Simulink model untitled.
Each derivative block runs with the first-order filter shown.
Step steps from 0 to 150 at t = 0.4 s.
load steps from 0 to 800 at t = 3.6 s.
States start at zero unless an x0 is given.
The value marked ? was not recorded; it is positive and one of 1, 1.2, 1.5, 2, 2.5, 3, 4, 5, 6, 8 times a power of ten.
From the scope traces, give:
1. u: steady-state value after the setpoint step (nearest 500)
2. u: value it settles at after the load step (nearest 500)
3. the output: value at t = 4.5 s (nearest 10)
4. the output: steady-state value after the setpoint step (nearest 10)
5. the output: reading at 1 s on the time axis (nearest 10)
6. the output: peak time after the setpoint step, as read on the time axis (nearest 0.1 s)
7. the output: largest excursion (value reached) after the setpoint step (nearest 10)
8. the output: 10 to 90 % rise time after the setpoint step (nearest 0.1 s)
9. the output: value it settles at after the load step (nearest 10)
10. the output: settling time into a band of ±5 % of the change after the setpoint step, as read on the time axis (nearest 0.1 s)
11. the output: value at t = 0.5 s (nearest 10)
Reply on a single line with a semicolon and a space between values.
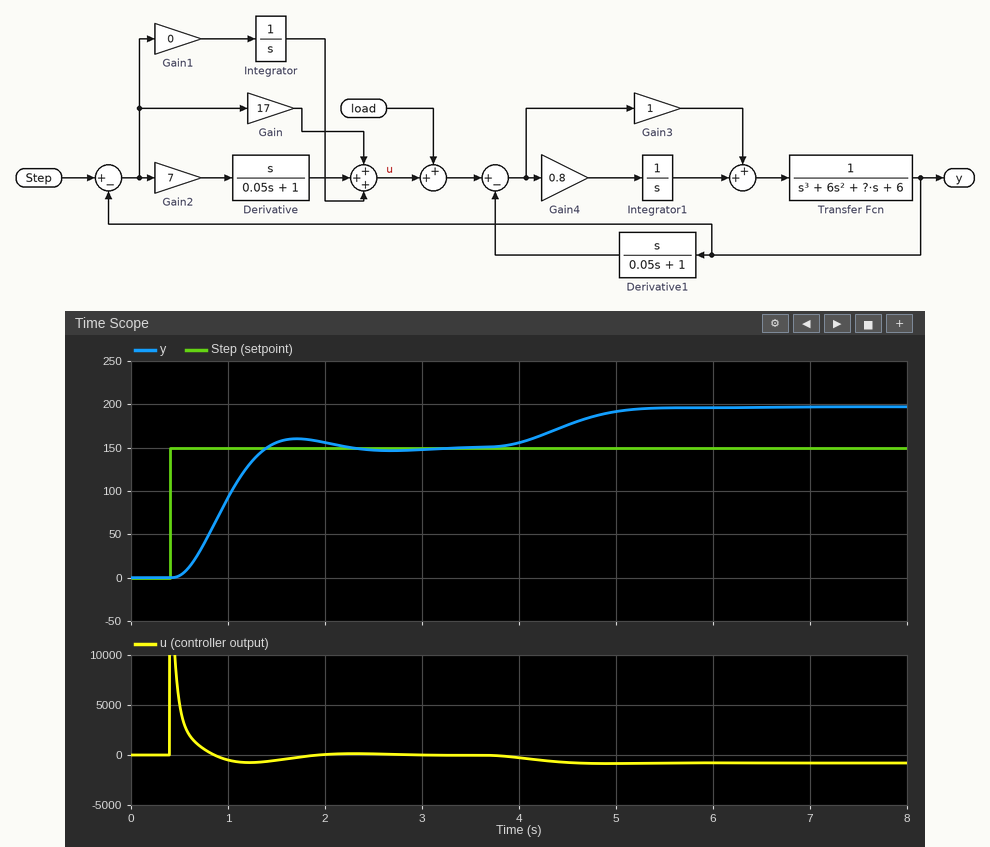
0; -1000; 180; 150; 90; 1.7 s; 160; 0.6 s; 200; 1.9 s; 0
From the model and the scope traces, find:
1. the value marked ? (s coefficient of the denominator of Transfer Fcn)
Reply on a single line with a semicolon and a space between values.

12
